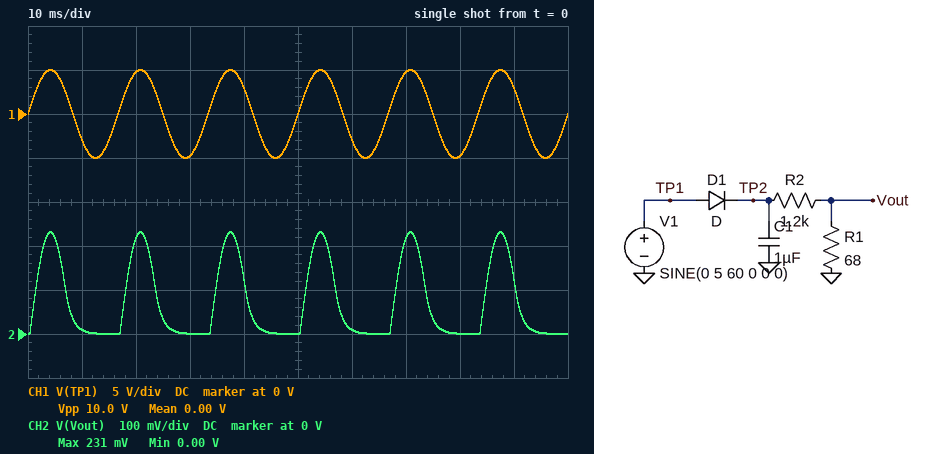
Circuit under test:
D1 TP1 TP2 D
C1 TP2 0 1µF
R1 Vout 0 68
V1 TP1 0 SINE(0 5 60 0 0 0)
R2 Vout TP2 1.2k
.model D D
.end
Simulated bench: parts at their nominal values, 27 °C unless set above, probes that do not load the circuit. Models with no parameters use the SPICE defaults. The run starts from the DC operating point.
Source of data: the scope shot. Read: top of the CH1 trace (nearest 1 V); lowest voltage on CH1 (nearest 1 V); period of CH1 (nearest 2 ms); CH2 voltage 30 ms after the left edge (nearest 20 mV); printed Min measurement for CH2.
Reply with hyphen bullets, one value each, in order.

- 5 V
- -5 V
- 16 ms
- 0 V
- 0.00 V
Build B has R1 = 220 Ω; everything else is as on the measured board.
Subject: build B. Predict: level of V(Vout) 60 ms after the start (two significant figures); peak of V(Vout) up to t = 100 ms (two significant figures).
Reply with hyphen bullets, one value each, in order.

- 35 mV
- 670 mV
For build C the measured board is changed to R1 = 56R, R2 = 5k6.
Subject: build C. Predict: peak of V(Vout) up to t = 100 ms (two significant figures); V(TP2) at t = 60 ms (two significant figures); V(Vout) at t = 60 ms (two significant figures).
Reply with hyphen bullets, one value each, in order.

- 43 mV
- 1.7 V
- 17 mV
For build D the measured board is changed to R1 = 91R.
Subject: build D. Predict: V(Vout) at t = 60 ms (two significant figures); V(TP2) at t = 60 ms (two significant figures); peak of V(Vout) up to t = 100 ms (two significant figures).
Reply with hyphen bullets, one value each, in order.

- 13 mV
- 180 mV
- 300 mV
